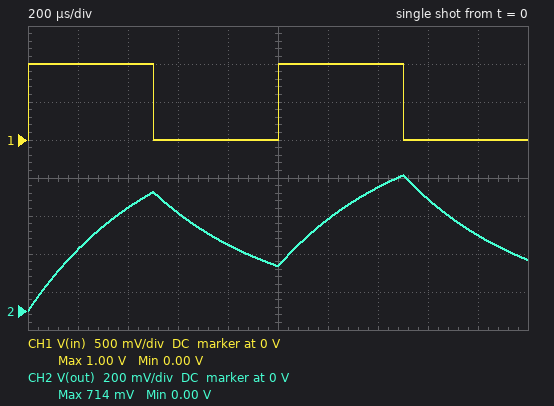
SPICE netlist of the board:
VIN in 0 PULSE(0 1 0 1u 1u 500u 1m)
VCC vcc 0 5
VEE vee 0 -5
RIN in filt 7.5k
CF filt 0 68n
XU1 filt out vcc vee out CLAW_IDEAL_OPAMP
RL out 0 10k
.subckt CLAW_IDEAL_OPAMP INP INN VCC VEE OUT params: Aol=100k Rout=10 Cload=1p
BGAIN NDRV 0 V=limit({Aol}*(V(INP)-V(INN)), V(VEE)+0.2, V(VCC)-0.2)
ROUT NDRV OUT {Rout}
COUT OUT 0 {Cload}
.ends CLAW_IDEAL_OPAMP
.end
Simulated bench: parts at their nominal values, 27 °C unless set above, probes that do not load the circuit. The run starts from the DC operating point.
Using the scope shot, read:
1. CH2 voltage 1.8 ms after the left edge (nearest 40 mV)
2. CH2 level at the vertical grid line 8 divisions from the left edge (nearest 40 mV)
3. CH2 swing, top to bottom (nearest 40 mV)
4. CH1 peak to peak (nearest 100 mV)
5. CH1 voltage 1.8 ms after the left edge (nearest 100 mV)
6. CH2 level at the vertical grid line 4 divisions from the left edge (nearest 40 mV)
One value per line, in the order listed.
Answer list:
400 mV
600 mV
720 mV
1.0 V
0 V
360 mV
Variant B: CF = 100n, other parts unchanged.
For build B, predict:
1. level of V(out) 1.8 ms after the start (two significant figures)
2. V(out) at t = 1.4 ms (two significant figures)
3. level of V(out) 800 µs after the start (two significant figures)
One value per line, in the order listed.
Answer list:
410 mV
560 mV
330 mV
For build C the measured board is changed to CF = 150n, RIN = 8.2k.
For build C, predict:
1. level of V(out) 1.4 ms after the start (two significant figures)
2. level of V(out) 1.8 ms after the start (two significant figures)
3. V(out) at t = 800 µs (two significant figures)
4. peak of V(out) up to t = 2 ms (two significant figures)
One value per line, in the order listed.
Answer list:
440 mV
380 mV
260 mV
480 mV
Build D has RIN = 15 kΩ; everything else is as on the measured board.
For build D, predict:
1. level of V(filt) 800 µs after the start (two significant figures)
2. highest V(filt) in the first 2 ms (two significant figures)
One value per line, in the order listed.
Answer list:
290 mV
530 mV
